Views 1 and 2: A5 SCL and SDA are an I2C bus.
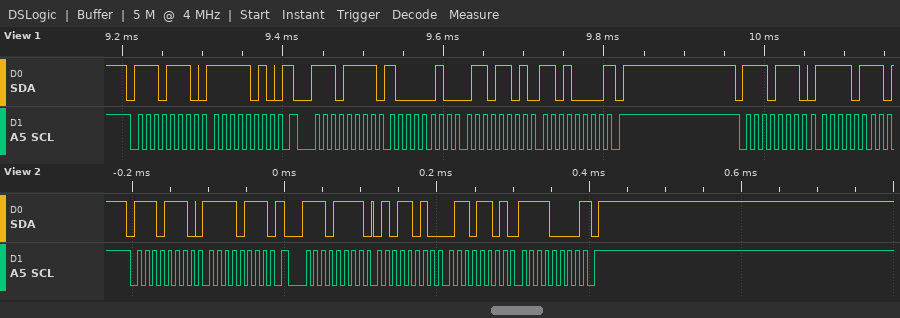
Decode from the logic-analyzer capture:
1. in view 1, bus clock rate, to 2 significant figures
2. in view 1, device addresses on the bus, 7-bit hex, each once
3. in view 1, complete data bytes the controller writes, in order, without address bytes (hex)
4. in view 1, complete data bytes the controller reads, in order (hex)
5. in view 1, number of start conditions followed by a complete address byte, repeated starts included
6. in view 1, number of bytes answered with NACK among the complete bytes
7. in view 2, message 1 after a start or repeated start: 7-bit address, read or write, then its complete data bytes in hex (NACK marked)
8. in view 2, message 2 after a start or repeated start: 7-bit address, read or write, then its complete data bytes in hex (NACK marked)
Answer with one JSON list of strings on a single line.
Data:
["100 kHz", "0x77", "FA F7", "82 6D D0", "3", "1", "0x77 write: F7", "0x77 read: 5A 6D F0 NACK"]
